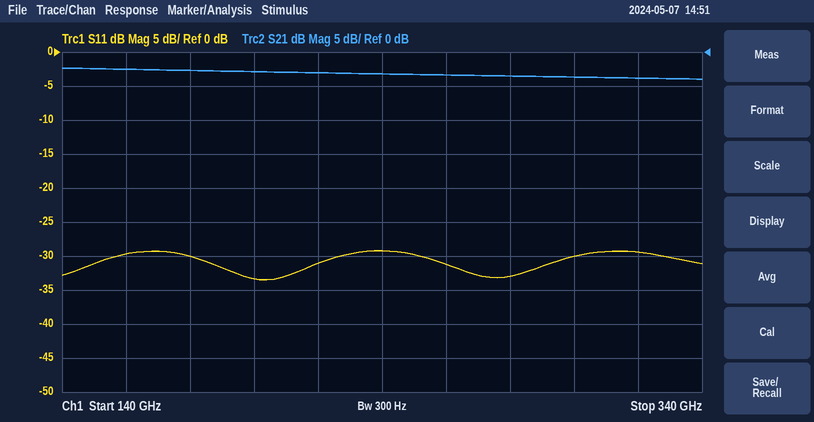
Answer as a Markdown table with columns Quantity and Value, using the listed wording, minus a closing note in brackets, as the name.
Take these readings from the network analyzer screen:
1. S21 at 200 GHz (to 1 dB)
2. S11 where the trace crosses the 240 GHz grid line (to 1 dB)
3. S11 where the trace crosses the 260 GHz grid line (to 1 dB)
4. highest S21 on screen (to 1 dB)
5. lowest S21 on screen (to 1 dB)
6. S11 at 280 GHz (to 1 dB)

| Quantity | Value |
|---|---|
| S21 at 200 GHz | -3 dB |
| S11 where the trace crosses the 240 GHz grid line | -29 dB |
| S11 where the trace crosses the 260 GHz grid line | -31 dB |
| highest S21 on screen | -2 dB |
| lowest S21 on screen | -4 dB |
| S11 at 280 GHz | -33 dB |
